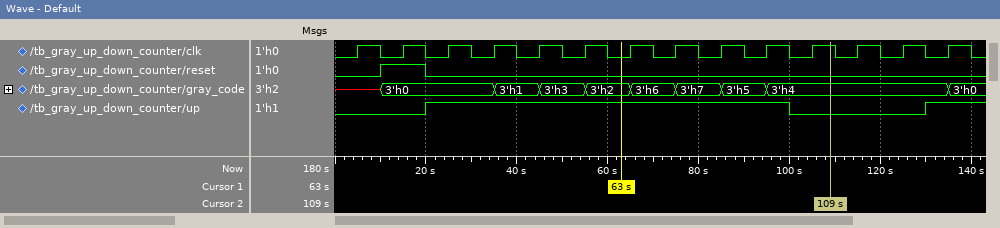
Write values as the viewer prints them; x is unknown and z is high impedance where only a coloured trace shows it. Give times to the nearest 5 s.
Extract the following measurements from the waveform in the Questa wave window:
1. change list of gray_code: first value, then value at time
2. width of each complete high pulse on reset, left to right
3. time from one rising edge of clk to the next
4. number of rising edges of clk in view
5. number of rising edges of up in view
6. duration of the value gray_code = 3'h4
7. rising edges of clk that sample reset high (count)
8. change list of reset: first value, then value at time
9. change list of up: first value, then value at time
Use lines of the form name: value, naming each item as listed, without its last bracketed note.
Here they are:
change list of gray_code: first value, then value at time: x, 3'h0 at 10 s, 3'h1 at 35 s, 3'h3 at 45 s, 3'h2 at 55 s, 3'h6 at 65 s, 3'h7 at 75 s, 3'h5 at 85 s, 3'h4 at 95 s, 3'h0 at 135 s
width of each complete high pulse on reset, left to right: 10 s
time from one rising edge of clk to the next: 10 s
number of rising edges of clk in view: 14
number of rising edges of up in view: 2
duration of the value gray_code = 3'h4: 40 s
rising edges of clk that sample reset high: 1
change list of reset: first value, then value at time: 0, 1 at 10 s, 0 at 20 s
change list of up: first value, then value at time: 0, 1 at 20 s, 0 at 100 s, 1 at 130 s
